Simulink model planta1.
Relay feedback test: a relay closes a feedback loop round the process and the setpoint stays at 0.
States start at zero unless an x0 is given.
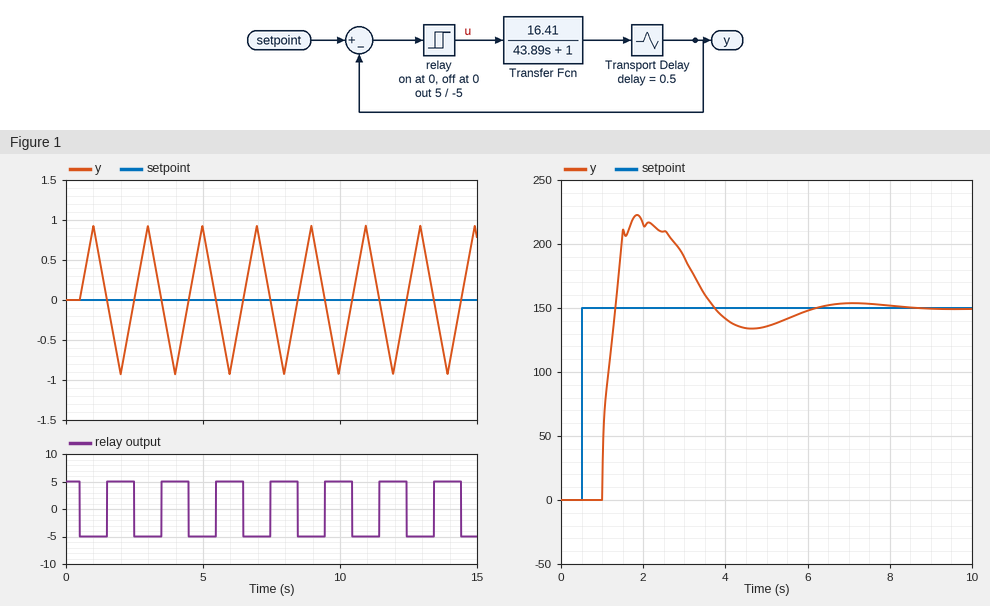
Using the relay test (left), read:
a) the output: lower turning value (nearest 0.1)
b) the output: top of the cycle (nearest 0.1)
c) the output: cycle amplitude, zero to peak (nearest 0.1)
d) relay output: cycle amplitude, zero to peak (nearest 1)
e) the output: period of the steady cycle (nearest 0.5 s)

-0.9
0.9
0.9
5
2.0 s
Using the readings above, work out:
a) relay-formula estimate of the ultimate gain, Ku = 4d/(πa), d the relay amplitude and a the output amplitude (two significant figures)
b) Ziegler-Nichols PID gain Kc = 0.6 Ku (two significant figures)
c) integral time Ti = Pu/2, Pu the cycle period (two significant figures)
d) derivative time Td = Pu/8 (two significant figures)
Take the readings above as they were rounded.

7.1
4.3
1.0 s
0.25 s
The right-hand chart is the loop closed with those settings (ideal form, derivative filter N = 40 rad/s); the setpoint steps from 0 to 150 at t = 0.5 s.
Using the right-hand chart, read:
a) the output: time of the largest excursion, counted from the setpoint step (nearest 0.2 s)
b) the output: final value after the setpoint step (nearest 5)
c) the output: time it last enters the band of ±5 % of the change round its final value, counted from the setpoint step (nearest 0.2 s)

1.4 s
150
5.0 s
